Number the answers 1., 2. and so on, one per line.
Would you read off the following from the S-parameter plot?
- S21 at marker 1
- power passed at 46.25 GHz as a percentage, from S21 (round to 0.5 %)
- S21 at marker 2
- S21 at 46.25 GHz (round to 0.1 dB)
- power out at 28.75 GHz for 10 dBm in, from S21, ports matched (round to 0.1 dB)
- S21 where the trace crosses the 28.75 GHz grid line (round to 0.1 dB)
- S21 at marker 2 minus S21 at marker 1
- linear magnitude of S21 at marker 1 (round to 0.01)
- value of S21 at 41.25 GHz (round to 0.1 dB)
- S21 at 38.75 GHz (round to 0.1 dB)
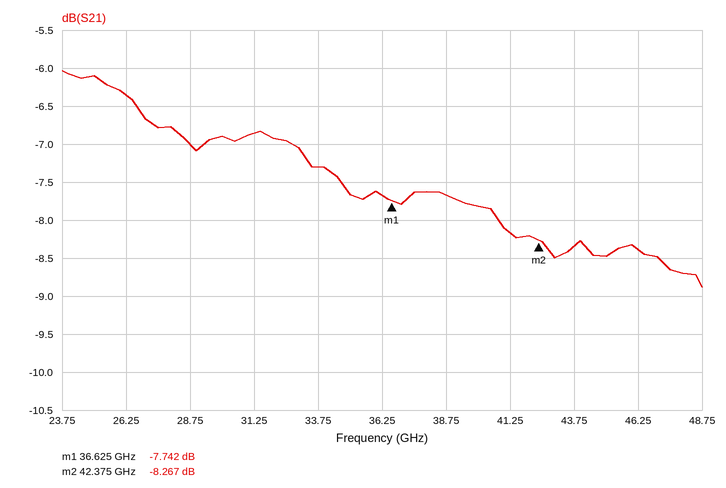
1. -7.742 dB
2. 14.5 %
3. -8.267 dB
4. -8.4 dB
5. 3.0 dBm
6. -7.0 dB
7. -0.525 dB
8. 0.41
9. -8.2 dB
10. -7.7 dB
